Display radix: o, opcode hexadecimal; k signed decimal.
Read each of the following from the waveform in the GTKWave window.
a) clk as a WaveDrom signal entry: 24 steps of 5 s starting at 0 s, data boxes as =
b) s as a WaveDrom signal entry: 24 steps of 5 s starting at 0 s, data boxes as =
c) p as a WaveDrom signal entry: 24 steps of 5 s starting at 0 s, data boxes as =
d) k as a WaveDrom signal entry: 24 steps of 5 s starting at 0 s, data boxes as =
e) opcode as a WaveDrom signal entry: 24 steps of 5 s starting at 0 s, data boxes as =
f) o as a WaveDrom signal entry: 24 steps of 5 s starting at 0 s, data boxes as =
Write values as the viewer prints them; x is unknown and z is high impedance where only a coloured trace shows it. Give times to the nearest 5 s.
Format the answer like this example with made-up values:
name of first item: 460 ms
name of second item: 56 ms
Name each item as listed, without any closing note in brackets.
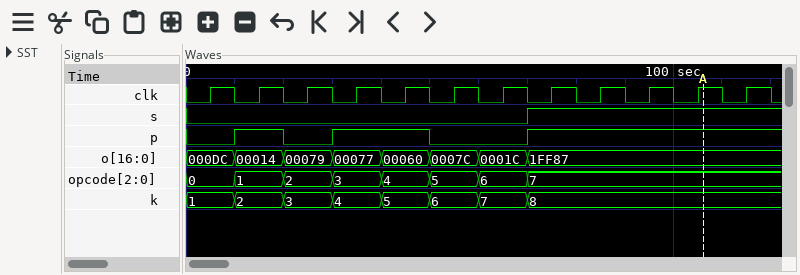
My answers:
clk as a WaveDrom signal entry: 24 steps of 5 s starting at 0 s, data boxes as =: {name: 'clk', wave: '010101010101010101010101'}
s as a WaveDrom signal entry: 24 steps of 5 s starting at 0 s, data boxes as =: {name: 's', wave: '0.............1.........'}
p as a WaveDrom signal entry: 24 steps of 5 s starting at 0 s, data boxes as =: {name: 'p', wave: '0.1.0.1...0...1.........'}
k as a WaveDrom signal entry: 24 steps of 5 s starting at 0 s, data boxes as =: {name: 'k', wave: '=.=.=.=.=.=.=.=.........', data: '1 2 3 4 5 6 7 8'}
opcode as a WaveDrom signal entry: 24 steps of 5 s starting at 0 s, data boxes as =: {name: 'opcode', wave: '=.=.=.=.=.=.=.=.........', data: '0 1 2 3 4 5 6 7'}
o as a WaveDrom signal entry: 24 steps of 5 s starting at 0 s, data boxes as =: {name: 'o', wave: '=.=.=.=.=.=.=.=.........', data: '000DC 00014 00079 00077 00060 0007C 0001C 1FF87'}
